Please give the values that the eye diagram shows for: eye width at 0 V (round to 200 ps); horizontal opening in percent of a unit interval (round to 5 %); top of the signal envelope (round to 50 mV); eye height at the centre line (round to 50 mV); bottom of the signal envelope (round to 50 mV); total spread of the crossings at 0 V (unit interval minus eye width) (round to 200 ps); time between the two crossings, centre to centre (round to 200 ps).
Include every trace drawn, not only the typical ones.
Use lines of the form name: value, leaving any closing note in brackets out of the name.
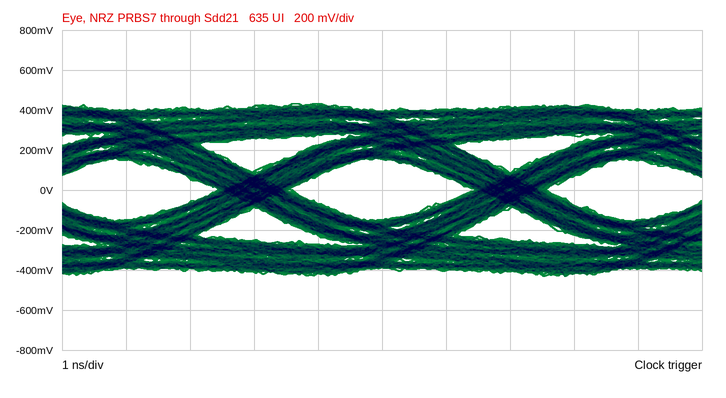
eye width at 0 V: 2.8 ns
horizontal opening in percent of a unit interval: 70 %
top of the signal envelope: 450 mV
eye height at the centre line: 300 mV
bottom of the signal envelope: -450 mV
total spread of the crossings at 0 V (unit interval minus eye width): 1.2 ns
time between the two crossings, centre to centre: 4.0 ns
